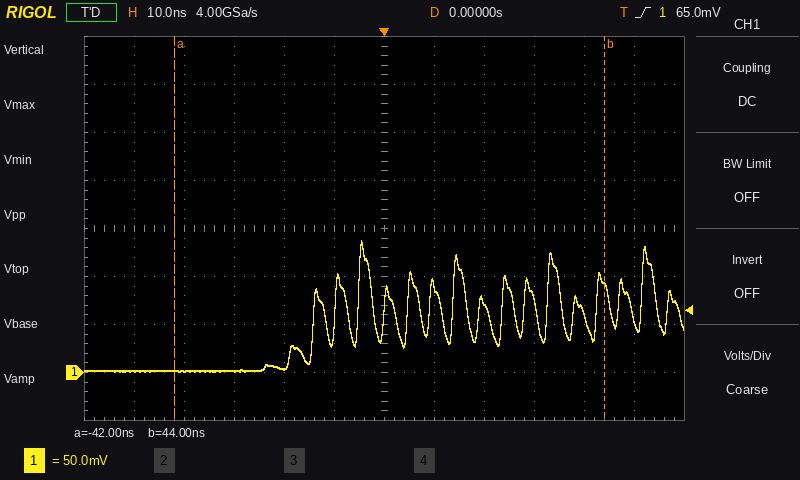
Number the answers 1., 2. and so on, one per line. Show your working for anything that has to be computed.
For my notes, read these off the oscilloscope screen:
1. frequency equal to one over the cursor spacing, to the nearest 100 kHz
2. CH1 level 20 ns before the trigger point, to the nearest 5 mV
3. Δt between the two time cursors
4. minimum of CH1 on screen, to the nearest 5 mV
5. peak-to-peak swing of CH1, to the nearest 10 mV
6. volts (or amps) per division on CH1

1. 1 / 86 ns ≈ 11.6 MHz
2. 5 mV
3. 44 ns − (-42 ns) = 86 ns
4. 0 mV
5. 140 mV
6. 50 mV
